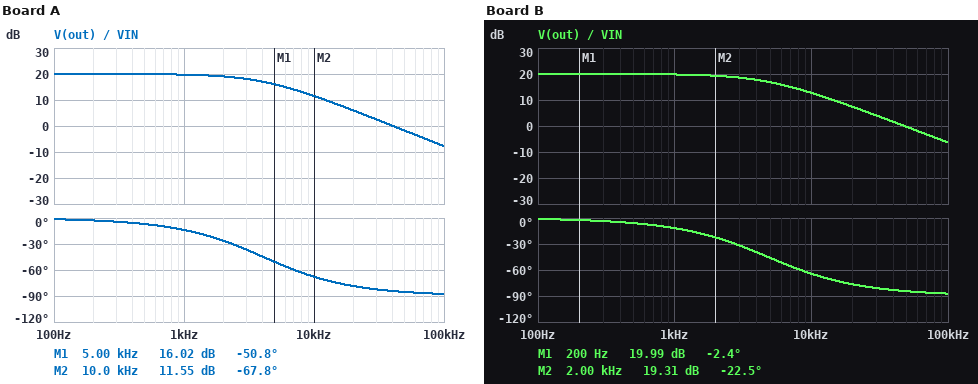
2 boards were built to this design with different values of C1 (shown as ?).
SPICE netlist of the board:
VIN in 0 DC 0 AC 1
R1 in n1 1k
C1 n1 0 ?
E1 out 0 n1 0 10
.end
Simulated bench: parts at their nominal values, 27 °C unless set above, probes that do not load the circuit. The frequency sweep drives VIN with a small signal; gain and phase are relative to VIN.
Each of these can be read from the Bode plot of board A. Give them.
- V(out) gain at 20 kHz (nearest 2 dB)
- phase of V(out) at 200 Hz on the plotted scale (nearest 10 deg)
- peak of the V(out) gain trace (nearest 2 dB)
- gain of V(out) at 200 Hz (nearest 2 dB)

6 dB
0 deg
20 dB
20 dB
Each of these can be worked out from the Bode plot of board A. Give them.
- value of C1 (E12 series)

39 nF
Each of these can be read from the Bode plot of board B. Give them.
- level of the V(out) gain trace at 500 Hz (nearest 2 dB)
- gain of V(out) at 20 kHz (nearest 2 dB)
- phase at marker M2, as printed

20 dB
8 dB
-22.5 deg
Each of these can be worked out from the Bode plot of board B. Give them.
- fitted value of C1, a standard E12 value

33 nF
